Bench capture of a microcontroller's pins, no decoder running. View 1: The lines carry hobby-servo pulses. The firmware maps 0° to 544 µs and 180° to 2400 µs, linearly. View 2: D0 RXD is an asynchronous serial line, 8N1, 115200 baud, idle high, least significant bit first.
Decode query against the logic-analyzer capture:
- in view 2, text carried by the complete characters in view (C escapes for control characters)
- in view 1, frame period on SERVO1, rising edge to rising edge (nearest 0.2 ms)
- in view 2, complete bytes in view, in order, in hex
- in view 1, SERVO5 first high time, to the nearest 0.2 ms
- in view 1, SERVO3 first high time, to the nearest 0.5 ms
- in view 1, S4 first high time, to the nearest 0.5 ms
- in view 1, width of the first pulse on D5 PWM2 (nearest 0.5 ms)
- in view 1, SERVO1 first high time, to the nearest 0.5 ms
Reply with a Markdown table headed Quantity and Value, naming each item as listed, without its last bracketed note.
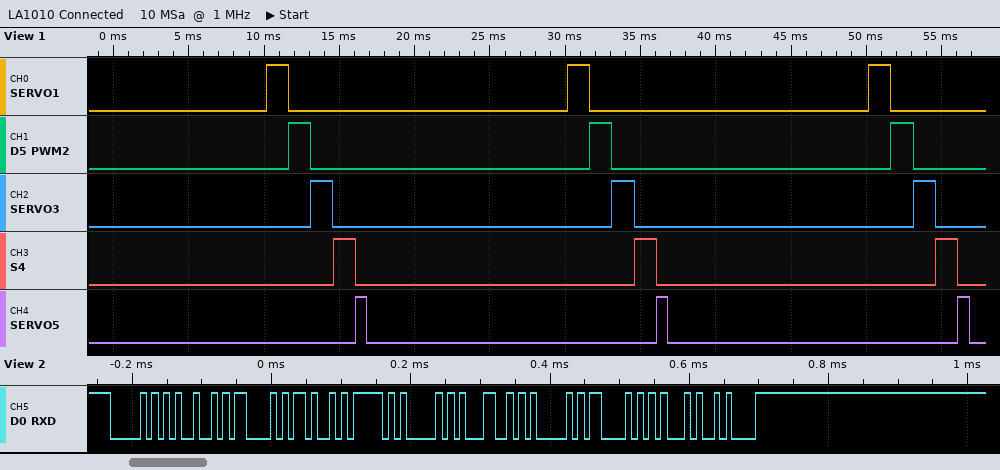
| Quantity | Value |
|---|---|
| in view 2, text carried by the complete characters in view | "PICK_PLACE\n" |
| in view 1, frame period on SERVO1, rising edge to rising edge | 20.0 ms |
| in view 2, complete bytes in view, in order, in hex | 50 49 43 4B 5F 50 4C 41 43 45 0A |
| in view 1, SERVO5 first high time, to the nearest 0.2 ms | 0.8 ms |
| in view 1, SERVO3 first high time, to the nearest 0.5 ms | 1.5 ms |
| in view 1, S4 first high time, to the nearest 0.5 ms | 1.5 ms |
| in view 1, width of the first pulse on D5 PWM2 | 1.5 ms |
| in view 1, SERVO1 first high time, to the nearest 0.5 ms | 1.5 ms |
